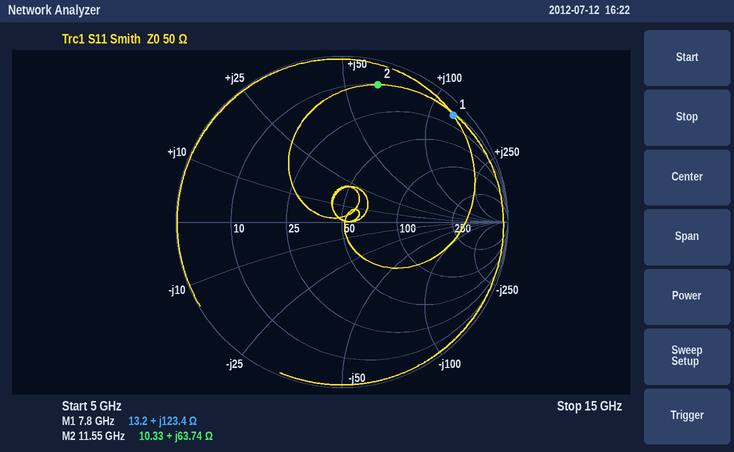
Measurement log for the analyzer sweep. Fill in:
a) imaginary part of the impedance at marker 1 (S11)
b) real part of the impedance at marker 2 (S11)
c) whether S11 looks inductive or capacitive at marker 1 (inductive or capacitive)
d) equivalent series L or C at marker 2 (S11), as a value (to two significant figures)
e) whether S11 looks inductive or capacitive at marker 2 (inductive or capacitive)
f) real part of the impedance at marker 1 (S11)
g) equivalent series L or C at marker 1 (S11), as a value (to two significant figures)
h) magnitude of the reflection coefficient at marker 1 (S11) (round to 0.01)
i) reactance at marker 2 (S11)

+123.4 Ω
10.33 Ω
inductive
880 pH
inductive
13.2 Ω
2.5 nH
0.93
+63.74 Ω
